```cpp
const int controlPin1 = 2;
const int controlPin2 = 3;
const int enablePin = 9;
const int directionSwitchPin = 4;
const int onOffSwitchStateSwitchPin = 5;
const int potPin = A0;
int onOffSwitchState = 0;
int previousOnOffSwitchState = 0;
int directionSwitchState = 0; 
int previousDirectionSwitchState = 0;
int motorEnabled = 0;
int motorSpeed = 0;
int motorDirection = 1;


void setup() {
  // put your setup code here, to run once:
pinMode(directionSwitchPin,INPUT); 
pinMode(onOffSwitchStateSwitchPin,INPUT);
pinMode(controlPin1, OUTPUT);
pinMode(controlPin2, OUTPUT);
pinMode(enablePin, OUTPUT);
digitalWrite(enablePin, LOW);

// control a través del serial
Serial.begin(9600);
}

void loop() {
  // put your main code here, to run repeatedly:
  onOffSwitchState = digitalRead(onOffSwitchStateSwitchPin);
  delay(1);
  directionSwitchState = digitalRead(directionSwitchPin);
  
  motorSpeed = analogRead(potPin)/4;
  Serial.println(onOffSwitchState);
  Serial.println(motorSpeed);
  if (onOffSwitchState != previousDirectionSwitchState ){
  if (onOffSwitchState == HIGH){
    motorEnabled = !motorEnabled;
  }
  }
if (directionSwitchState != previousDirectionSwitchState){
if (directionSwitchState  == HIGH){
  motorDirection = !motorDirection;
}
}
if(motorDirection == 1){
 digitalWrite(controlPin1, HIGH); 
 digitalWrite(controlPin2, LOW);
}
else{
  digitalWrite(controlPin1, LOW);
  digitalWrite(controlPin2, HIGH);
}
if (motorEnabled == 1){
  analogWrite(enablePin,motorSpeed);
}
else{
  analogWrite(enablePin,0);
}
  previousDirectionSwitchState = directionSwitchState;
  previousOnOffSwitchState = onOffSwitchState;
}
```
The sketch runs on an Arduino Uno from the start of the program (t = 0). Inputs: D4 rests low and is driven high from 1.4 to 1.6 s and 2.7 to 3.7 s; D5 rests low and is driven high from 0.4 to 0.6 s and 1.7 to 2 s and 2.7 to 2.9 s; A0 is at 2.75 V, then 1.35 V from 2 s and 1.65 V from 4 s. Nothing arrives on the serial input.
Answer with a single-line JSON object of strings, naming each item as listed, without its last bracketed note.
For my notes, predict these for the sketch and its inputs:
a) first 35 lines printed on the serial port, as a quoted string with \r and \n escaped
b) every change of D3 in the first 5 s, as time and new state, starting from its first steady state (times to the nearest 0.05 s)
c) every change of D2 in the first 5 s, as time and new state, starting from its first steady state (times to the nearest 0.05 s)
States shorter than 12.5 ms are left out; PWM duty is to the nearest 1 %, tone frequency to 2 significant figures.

{"first 35 lines printed on the serial port, as a quoted string with \\r and \\n escaped": "\"0\\r\\n140\\r\\n0\\r\\n140\\r\\n0\\r\\n140\\r\\n0\\r\\n140\\r\\n0\\r\\n140\\r\\n0\\r\\n140\\r\\n0\\r\\n140\\r\\n0\\r\\n140\\r\\n0\\r\\n140\\r\\n0\\r\\n140\\r\\n0\\r\\n140\\r\\n0\\r\\n140\\r\\n0\\r\\n140\\r\\n0\\r\\n140\\r\\n0\\r\\n140\\r\\n0\\r\\n140\\r\\n0\\r\\n140\\r\\n0\\r\\n\"", "every change of D3 in the first 5 s, as time and new state, starting from its first steady state": "0 s low; 1.4 s high; 2.7 s low", "every change of D2 in the first 5 s, as time and new state, starting from its first steady state": "0 s high; 1.4 s low; 2.7 s high"}
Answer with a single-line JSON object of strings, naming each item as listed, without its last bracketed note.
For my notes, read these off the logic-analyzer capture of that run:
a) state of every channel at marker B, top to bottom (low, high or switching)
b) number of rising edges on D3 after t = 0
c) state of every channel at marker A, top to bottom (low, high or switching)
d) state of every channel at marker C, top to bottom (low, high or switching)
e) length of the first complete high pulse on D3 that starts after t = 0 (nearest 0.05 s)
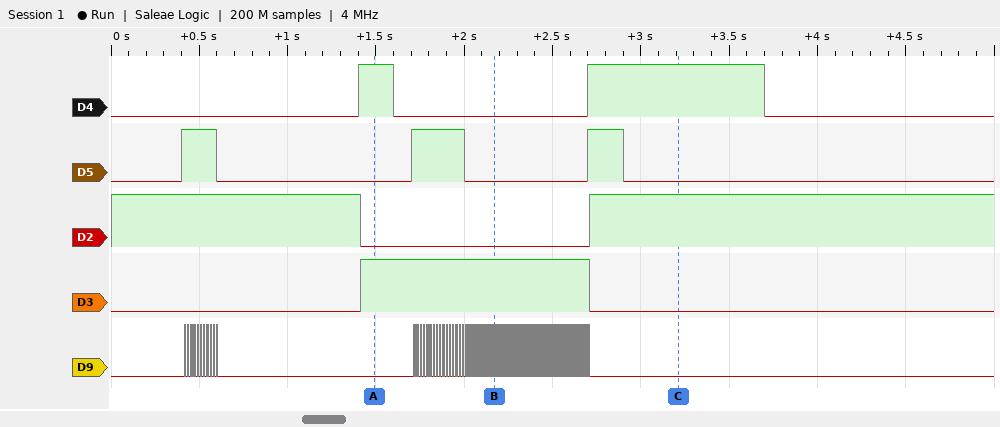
{"state of every channel at marker B, top to bottom": "D4 low, D5 low, D2 low, D3 high, D9 switching", "number of rising edges on D3 after t = 0": "1", "state of every channel at marker A, top to bottom": "D4 high, D5 low, D2 low, D3 high, D9 low", "state of every channel at marker C, top to bottom": "D4 high, D5 low, D2 high, D3 low, D9 low", "length of the first complete high pulse on D3 that starts after t = 0": "1.30 s"}
